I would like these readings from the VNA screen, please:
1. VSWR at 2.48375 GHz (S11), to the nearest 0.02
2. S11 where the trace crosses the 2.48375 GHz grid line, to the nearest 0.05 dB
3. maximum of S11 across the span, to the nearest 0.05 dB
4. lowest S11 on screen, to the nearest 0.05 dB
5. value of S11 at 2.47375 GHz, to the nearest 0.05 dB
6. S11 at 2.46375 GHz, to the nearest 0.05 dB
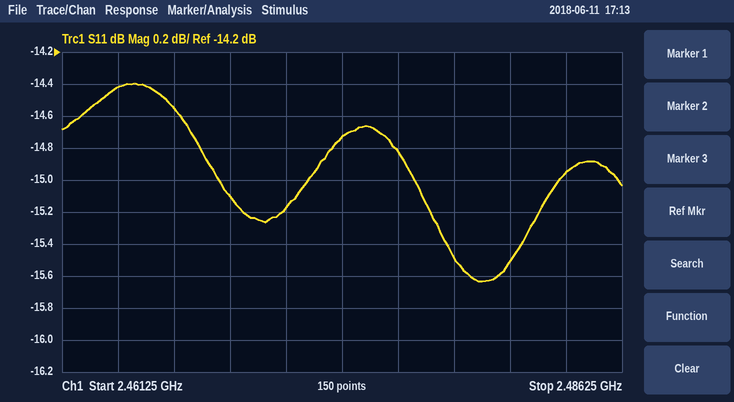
1.44
-14.95 dB
-14.40 dB
-15.65 dB
-14.75 dB
-14.40 dB
